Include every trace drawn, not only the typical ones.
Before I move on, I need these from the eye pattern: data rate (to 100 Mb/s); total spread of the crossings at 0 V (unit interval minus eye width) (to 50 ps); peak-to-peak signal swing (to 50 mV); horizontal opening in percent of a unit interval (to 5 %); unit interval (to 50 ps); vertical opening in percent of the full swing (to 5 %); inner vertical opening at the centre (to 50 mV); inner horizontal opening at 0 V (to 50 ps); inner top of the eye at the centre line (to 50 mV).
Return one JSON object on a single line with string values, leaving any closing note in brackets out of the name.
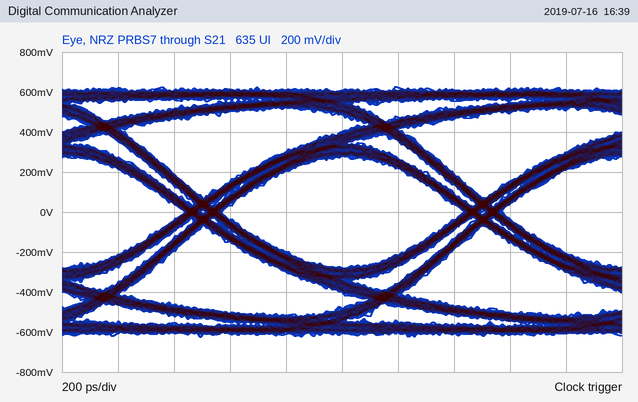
{"data rate": "1.0 Gb/s", "total spread of the crossings at 0 V (unit interval minus eye width)": "150 ps", "peak-to-peak signal swing": "1.25 V", "horizontal opening in percent of a unit interval": "85 %", "unit interval": "1.00 ns", "vertical opening in percent of the full swing": "45 %", "inner vertical opening at the centre": "550 mV", "inner horizontal opening at 0 V": "850 ps", "inner top of the eye at the centre line": "300 mV"}
